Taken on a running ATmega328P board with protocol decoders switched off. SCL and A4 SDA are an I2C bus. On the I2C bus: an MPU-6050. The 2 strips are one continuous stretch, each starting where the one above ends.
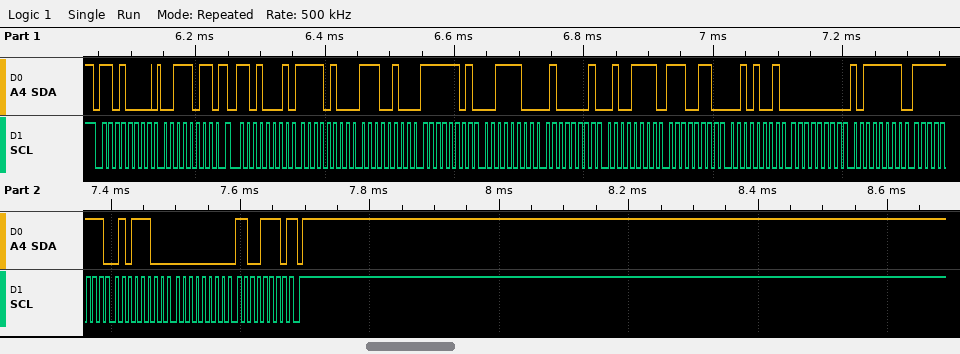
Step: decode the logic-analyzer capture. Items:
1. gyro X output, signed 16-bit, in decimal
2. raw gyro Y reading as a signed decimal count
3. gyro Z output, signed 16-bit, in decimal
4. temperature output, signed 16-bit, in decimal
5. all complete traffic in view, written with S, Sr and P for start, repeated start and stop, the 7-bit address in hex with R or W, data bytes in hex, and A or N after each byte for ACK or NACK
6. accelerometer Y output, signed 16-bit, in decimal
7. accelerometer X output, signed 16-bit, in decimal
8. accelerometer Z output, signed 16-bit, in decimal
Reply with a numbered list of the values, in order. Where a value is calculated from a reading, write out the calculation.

1. 0x00BF = 191
2. 0xFF5C = -164
3. 0x00CE = 206
4. 0xE629 = -6615
5. S 68W A 3B A Sr 68R A F4 A E4 A FD A 3C A 41 A 4F A E6 A 29 A 00 A BF A FF A 5C A 00 A CE N P
6. 0xFD3C = -708
7. 0xF4E4 = -2844
8. 0x414F = 16719
